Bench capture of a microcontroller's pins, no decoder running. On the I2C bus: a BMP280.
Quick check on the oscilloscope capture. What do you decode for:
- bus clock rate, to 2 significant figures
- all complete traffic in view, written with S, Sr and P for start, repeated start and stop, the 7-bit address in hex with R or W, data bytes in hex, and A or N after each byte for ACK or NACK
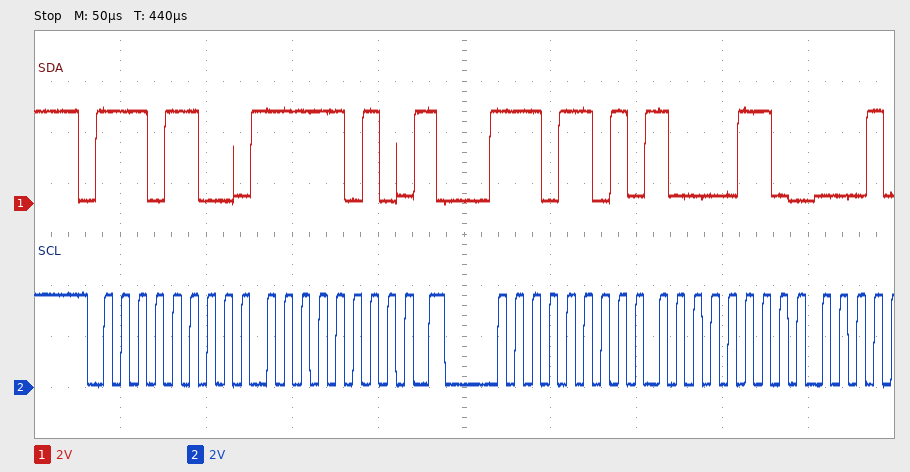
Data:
100 kHz
S 76W A FA A Sr 76R A 86 A
